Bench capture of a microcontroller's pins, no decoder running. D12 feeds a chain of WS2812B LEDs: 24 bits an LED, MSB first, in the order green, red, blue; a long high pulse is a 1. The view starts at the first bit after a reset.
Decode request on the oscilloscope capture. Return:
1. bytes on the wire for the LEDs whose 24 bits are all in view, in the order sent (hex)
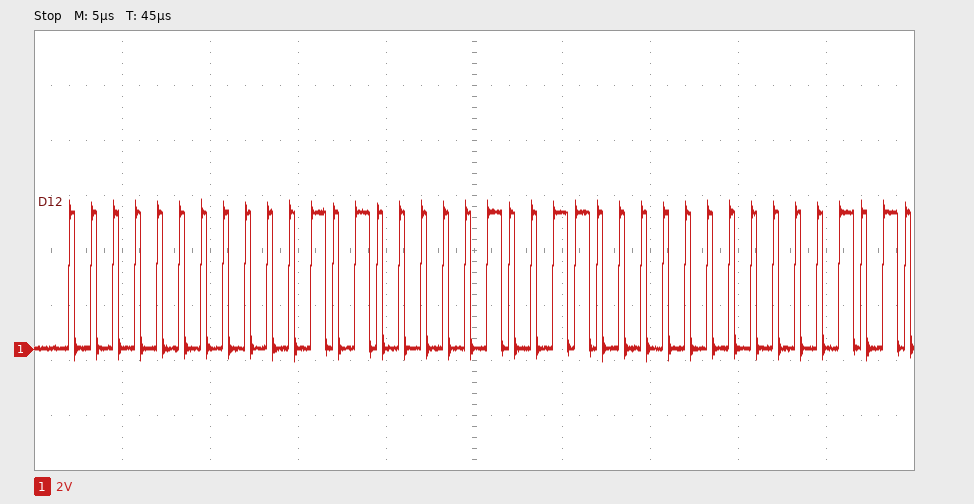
00 14 13
